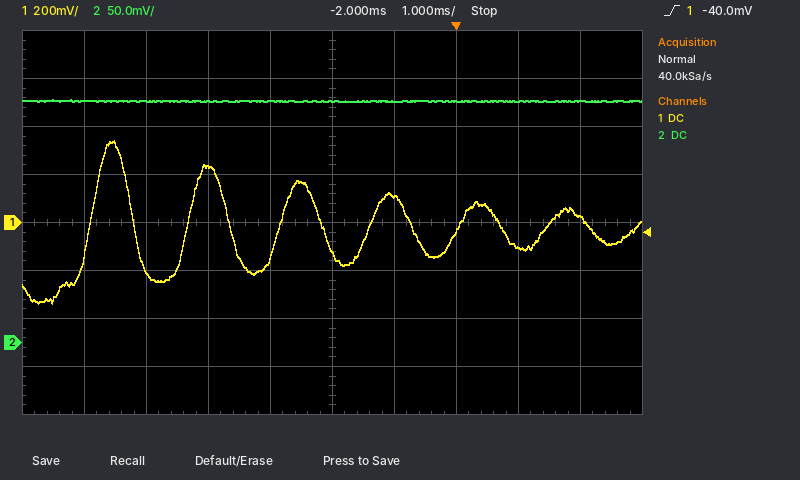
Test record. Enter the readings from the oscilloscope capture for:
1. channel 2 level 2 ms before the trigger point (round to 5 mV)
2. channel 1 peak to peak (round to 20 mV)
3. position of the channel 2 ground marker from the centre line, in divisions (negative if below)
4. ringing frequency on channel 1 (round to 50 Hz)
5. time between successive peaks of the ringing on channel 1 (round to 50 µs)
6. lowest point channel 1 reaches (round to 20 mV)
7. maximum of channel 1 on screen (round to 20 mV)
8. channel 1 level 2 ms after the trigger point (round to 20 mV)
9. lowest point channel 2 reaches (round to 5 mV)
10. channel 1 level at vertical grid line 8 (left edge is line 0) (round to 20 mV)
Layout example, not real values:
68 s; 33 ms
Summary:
250 mV; 680 mV; -2.5 div; 700 Hz; 1.45 ms; -340 mV; 340 mV; 20 mV; 250 mV; -100 mV
